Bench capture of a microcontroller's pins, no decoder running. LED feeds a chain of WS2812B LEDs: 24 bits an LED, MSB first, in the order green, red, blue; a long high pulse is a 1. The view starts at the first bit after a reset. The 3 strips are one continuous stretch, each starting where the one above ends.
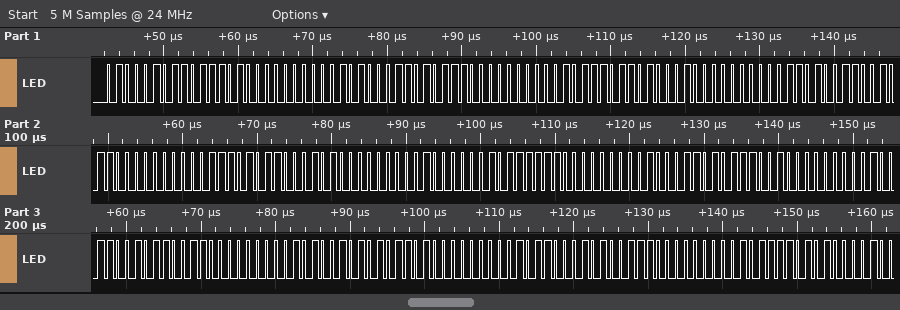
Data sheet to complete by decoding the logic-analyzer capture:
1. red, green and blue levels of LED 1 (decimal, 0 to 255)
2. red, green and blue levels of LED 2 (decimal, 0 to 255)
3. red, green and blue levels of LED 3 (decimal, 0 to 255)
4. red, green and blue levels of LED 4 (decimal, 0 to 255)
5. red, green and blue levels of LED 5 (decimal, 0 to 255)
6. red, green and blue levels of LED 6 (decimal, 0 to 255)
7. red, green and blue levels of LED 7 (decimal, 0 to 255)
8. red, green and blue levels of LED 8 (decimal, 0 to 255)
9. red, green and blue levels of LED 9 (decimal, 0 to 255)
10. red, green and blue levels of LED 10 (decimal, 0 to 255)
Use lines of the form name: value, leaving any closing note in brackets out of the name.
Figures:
red, green and blue levels of LED 1: 186, 69, 0
red, green and blue levels of LED 2: 174, 81, 0
red, green and blue levels of LED 3: 162, 93, 0
red, green and blue levels of LED 4: 150, 105, 0
red, green and blue levels of LED 5: 138, 117, 0
red, green and blue levels of LED 6: 126, 129, 0
red, green and blue levels of LED 7: 114, 141, 0
red, green and blue levels of LED 8: 102, 153, 0
red, green and blue levels of LED 9: 90, 165, 0
red, green and blue levels of LED 10: 78, 177, 0
